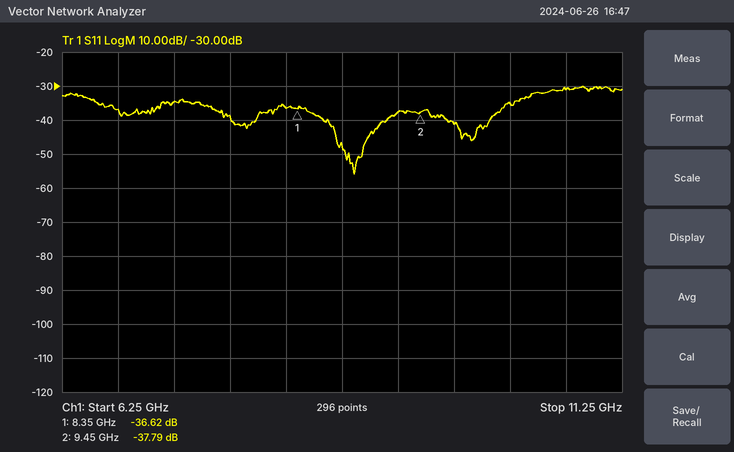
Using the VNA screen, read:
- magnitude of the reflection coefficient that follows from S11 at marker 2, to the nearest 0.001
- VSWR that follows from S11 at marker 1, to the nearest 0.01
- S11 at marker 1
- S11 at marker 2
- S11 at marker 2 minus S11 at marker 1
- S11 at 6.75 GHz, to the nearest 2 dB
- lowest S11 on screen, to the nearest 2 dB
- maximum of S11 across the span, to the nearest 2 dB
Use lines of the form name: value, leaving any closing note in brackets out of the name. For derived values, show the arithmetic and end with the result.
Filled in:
magnitude of the reflection coefficient that follows from S11 at marker 2, to the nearest 0.001: 10^(-37.79/20) ≈ 0.013
VSWR that follows from S11 at marker 1, to the nearest 0.01: (1 + 0.0148)/(1 − 0.0148) ≈ 1.03
S11 at marker 1: -36.62 dB
S11 at marker 2: -37.79 dB
S11 at marker 2 minus S11 at marker 1: -37.79 − (-36.62) = -1.17 dB
S11 at 6.75 GHz, to the nearest 2 dB: -36 dB
lowest S11 on screen, to the nearest 2 dB: -56 dB
maximum of S11 across the span, to the nearest 2 dB: -30 dB
